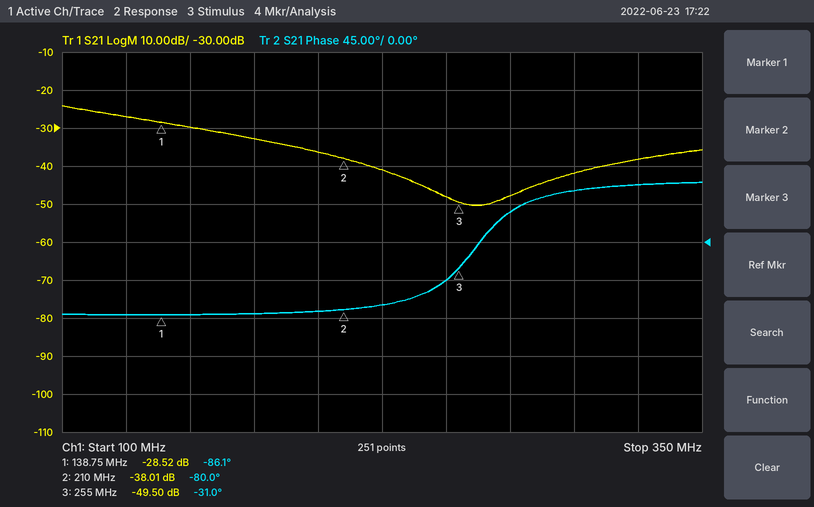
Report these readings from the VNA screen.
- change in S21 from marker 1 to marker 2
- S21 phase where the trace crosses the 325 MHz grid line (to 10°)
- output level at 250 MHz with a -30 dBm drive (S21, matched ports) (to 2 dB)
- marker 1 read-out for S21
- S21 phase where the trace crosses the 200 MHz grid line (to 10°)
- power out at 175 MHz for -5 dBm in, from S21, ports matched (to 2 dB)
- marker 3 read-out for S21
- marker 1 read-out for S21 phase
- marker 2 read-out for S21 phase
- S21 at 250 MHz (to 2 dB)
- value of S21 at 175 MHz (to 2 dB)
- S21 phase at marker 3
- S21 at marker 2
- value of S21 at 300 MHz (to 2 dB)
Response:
-9.49 dB
70°
-78 dBm
-28.52 dB
-80°
-38 dBm
-49.50 dB
-86.1°
-80.0°
-48 dB
-32 dB
-31.0°
-38.01 dB
-42 dB
